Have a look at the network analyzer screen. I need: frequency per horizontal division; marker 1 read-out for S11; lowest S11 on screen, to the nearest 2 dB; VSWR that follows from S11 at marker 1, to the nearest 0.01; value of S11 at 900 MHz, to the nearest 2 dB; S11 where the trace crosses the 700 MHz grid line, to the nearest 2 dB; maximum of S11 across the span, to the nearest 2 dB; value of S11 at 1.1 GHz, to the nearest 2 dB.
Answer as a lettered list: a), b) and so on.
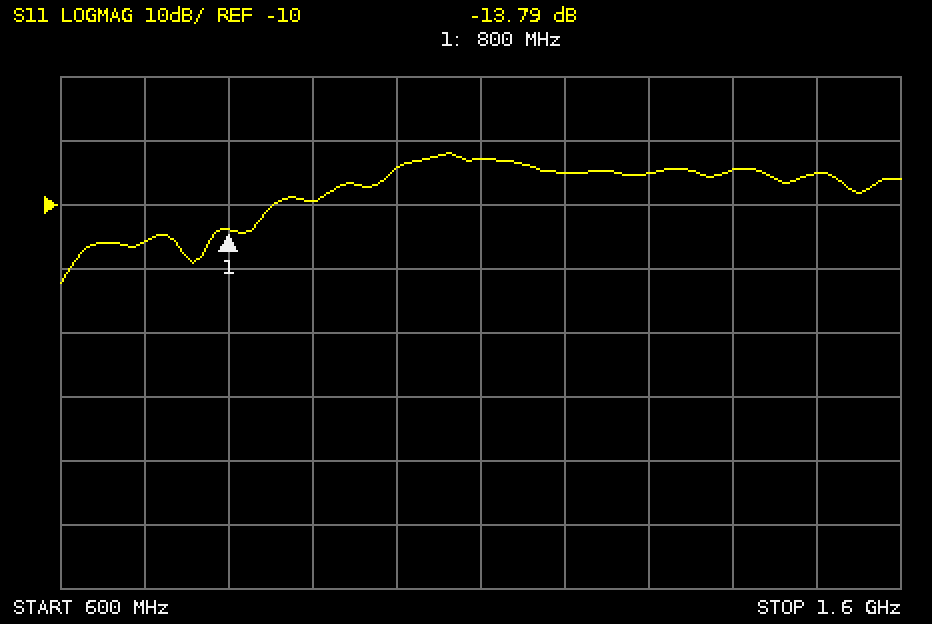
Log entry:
a) 100 MHz
b) -13.79 dB
c) -22 dB
d) 1.51
e) -10 dB
f) -16 dB
g) -2 dB
h) -2 dB
